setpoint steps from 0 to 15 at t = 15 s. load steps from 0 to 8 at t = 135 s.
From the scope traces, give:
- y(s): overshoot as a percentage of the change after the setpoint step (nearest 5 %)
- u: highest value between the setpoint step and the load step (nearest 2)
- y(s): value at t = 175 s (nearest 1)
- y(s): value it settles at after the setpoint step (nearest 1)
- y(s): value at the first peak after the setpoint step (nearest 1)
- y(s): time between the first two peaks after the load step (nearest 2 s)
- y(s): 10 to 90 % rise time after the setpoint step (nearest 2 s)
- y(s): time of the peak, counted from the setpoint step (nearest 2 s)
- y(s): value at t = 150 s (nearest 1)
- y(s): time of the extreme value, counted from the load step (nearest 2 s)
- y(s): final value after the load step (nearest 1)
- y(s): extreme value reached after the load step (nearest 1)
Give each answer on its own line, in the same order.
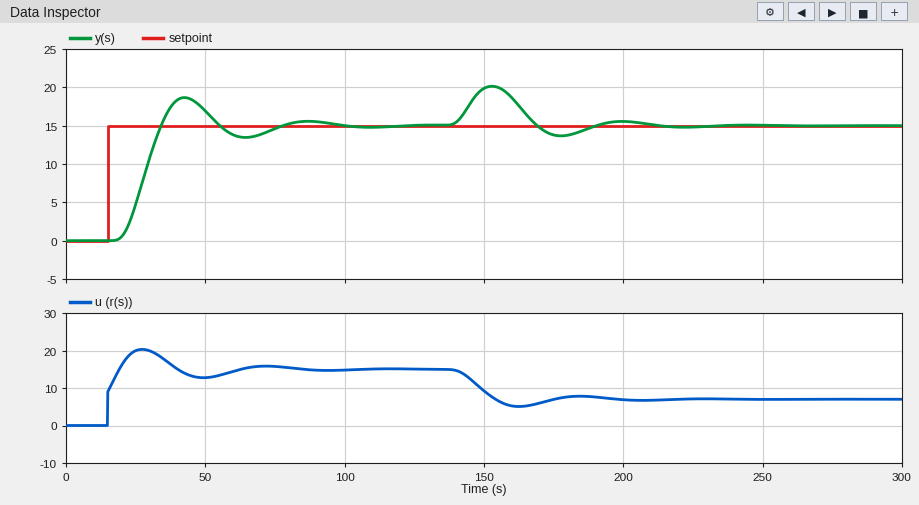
25 %
20
14
15
19
46 s
10 s
28 s
20
18 s
15
20
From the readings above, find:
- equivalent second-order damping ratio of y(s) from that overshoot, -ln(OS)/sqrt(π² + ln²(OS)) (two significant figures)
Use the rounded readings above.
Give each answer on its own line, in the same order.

0.40
